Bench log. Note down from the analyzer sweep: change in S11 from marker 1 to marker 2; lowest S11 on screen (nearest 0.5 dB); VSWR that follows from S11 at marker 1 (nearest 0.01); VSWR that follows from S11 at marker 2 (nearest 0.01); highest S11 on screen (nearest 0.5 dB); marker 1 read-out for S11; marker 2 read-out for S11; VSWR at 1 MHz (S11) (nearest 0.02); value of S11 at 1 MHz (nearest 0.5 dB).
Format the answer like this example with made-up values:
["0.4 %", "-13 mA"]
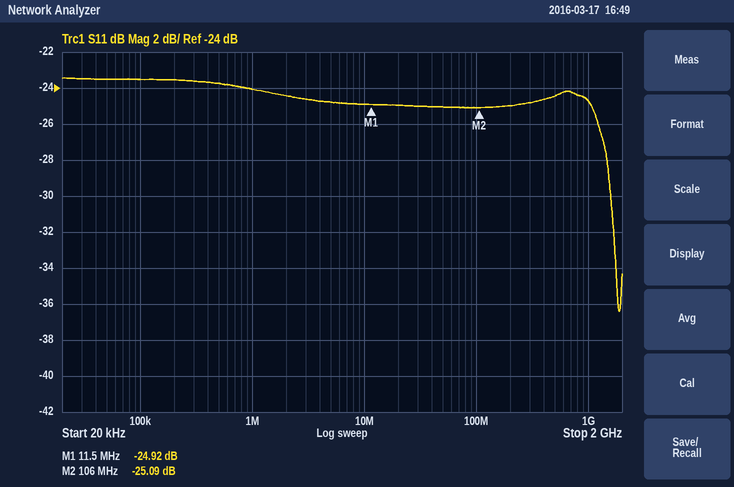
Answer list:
["-0.17 dB", "-36.5 dB", "1.12", "1.12", "-23.5 dB", "-24.92 dB", "-25.09 dB", "1.14", "-24.0 dB"]
